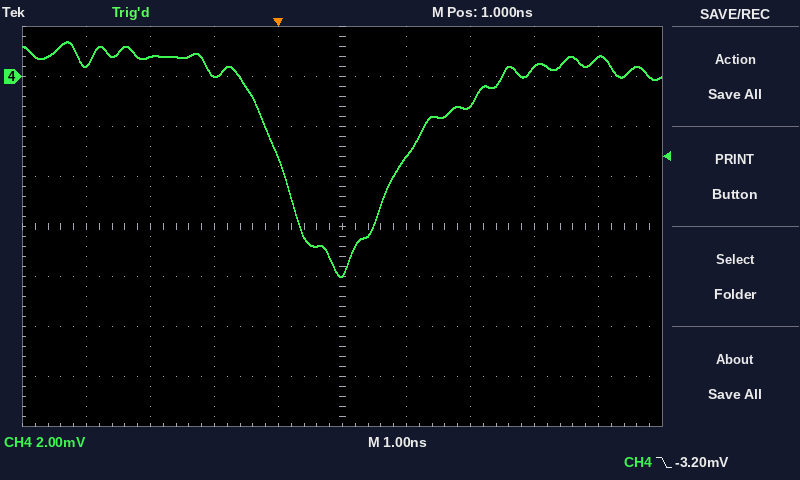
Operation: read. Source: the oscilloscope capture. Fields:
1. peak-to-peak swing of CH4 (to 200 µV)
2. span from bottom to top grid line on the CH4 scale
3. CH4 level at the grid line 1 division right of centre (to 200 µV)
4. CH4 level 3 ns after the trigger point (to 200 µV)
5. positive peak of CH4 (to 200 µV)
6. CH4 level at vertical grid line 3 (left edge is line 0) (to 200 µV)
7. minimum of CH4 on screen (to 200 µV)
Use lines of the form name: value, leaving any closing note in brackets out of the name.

peak-to-peak swing of CH4: 9.4 mV
span from bottom to top grid line on the CH4 scale: 16 mV
CH4 level at the grid line 1 division right of centre: -3.2 mV
CH4 level 3 ns after the trigger point: -1.2 mV
positive peak of CH4: 1.4 mV
CH4 level at vertical grid line 3 (left edge is line 0): 0.0 mV
minimum of CH4 on screen: -8.0 mV
